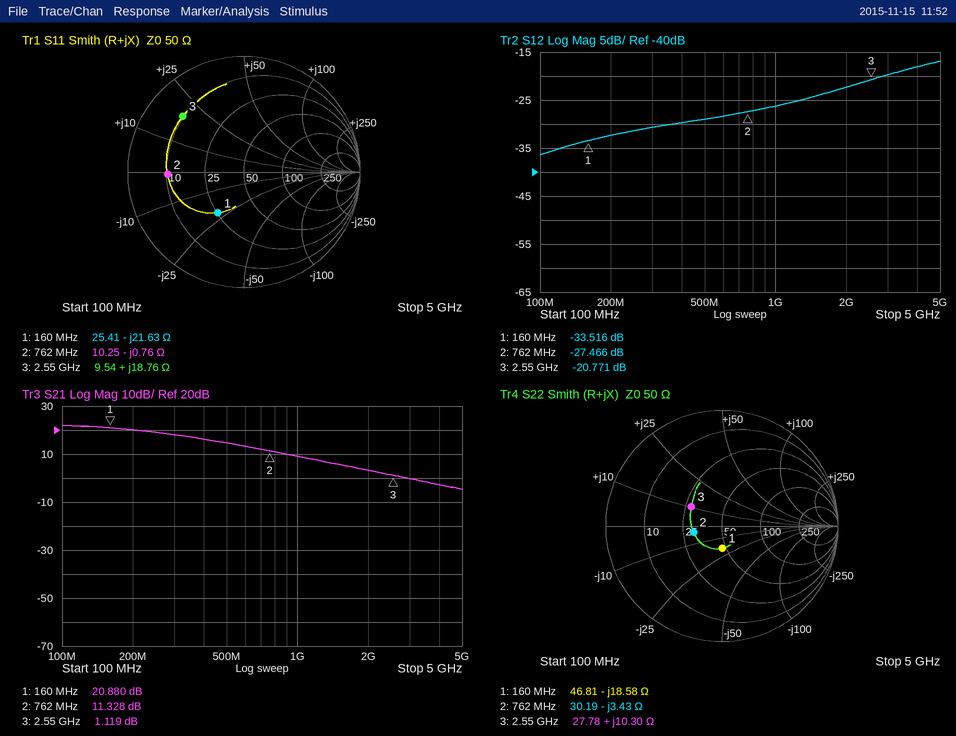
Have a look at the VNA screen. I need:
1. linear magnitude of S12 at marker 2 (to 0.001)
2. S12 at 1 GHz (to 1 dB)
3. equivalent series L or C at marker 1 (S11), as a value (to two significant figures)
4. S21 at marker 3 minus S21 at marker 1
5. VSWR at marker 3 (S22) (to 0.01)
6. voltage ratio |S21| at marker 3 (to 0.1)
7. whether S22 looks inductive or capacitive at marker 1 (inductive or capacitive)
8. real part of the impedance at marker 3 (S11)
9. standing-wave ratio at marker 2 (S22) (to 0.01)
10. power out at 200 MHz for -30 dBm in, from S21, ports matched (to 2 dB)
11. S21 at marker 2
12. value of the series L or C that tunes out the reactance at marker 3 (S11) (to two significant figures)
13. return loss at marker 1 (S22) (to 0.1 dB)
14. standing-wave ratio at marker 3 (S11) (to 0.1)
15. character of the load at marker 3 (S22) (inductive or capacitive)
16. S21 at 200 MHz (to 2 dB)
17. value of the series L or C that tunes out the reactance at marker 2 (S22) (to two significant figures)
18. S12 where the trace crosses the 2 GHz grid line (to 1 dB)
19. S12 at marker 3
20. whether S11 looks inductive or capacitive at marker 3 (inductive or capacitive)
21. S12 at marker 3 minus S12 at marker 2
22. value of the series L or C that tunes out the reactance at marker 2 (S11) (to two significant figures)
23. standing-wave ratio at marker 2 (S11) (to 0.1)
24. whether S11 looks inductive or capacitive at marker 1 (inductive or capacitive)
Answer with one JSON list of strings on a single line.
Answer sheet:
["0.042", "-26 dB", "46 pF", "-19.761 dB", "1.91", "1.1", "capacitive", "9.54 Ω", "1.67", "-10 dBm", "11.328 dB", "3.3 pF", "14.4 dB", "6.0", "inductive", "20 dB", "720 pH", "-22 dB", "-20.771 dB", "inductive", "6.695 dB", "160 pH", "4.9", "capacitive"]
